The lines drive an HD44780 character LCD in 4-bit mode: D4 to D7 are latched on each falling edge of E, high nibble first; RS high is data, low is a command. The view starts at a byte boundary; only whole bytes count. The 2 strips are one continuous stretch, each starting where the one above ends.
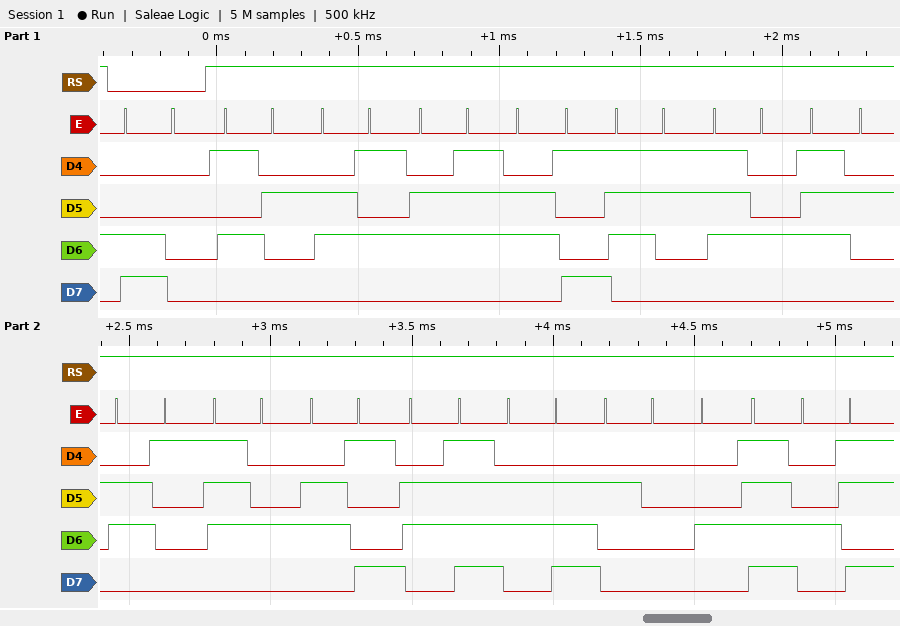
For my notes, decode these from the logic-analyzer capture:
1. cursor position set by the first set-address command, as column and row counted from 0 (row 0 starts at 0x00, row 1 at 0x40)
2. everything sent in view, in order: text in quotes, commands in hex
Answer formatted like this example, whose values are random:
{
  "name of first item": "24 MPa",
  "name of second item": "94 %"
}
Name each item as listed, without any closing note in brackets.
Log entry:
{
  "cursor position set by the first set-address command, as column and row counted from 0": "column 0, row 1",
  "everything sent in view, in order: text in quotes, commands in hex": "0xC0 \"Registration OK\""
}
